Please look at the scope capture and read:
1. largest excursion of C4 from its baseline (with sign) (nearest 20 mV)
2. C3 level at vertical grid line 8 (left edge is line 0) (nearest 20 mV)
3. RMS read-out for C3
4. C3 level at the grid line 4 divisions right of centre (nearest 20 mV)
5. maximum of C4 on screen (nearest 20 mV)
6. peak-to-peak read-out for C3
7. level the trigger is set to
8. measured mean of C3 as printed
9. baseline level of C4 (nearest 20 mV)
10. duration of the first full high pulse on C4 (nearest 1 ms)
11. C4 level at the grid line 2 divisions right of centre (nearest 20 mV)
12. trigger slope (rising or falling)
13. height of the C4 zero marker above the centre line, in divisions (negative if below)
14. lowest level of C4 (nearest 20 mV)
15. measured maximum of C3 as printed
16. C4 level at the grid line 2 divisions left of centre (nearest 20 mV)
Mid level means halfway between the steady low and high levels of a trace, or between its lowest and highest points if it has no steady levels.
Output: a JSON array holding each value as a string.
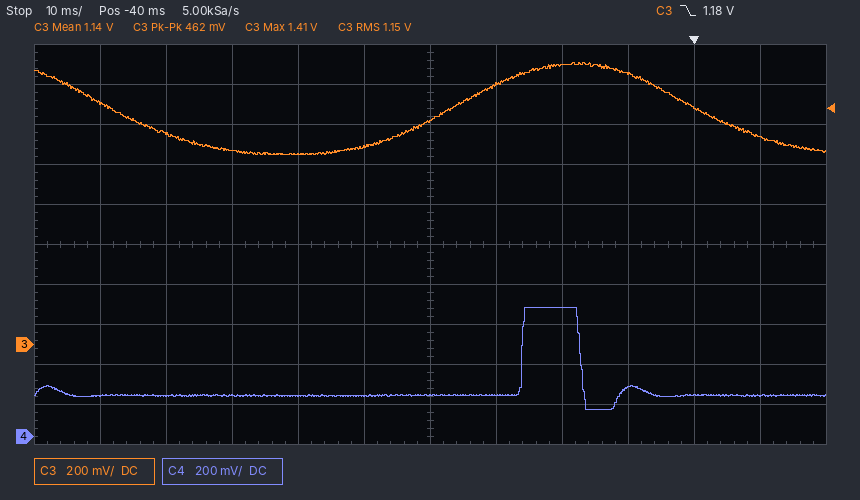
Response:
["+440 mV", "1.40 V", "1.15 V", "1.18 V", "640 mV", "462 mV", "1.18 V", "1.14 V", "200 mV", "9 ms", "640 mV", "falling", "-4.8 div", "140 mV", "1.41 V", "200 mV"]
